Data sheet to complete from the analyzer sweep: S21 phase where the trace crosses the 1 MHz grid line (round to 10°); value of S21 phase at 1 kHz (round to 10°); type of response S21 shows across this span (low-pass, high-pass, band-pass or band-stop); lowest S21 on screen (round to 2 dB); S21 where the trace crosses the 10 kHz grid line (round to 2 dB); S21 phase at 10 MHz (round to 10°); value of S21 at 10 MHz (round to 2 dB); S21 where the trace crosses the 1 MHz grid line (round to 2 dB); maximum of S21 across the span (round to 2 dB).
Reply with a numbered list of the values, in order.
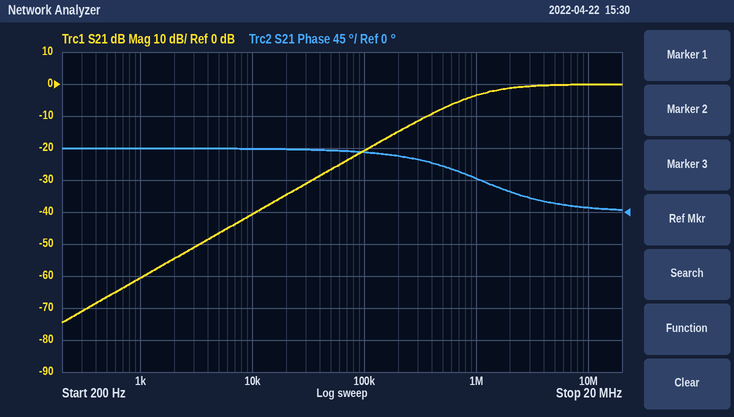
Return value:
1. 50°
2. 90°
3. high-pass
4. -74 dB
5. -40 dB
6. 10°
7. 0 dB
8. -4 dB
9. 0 dB
